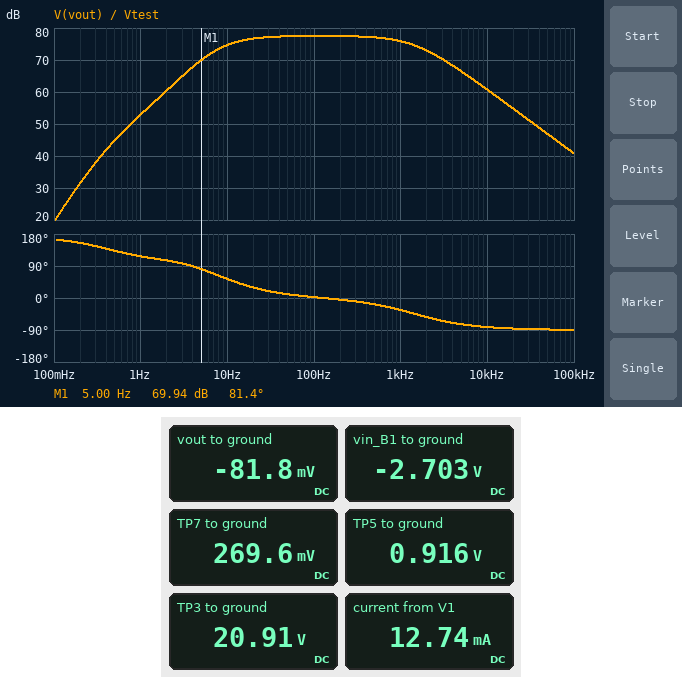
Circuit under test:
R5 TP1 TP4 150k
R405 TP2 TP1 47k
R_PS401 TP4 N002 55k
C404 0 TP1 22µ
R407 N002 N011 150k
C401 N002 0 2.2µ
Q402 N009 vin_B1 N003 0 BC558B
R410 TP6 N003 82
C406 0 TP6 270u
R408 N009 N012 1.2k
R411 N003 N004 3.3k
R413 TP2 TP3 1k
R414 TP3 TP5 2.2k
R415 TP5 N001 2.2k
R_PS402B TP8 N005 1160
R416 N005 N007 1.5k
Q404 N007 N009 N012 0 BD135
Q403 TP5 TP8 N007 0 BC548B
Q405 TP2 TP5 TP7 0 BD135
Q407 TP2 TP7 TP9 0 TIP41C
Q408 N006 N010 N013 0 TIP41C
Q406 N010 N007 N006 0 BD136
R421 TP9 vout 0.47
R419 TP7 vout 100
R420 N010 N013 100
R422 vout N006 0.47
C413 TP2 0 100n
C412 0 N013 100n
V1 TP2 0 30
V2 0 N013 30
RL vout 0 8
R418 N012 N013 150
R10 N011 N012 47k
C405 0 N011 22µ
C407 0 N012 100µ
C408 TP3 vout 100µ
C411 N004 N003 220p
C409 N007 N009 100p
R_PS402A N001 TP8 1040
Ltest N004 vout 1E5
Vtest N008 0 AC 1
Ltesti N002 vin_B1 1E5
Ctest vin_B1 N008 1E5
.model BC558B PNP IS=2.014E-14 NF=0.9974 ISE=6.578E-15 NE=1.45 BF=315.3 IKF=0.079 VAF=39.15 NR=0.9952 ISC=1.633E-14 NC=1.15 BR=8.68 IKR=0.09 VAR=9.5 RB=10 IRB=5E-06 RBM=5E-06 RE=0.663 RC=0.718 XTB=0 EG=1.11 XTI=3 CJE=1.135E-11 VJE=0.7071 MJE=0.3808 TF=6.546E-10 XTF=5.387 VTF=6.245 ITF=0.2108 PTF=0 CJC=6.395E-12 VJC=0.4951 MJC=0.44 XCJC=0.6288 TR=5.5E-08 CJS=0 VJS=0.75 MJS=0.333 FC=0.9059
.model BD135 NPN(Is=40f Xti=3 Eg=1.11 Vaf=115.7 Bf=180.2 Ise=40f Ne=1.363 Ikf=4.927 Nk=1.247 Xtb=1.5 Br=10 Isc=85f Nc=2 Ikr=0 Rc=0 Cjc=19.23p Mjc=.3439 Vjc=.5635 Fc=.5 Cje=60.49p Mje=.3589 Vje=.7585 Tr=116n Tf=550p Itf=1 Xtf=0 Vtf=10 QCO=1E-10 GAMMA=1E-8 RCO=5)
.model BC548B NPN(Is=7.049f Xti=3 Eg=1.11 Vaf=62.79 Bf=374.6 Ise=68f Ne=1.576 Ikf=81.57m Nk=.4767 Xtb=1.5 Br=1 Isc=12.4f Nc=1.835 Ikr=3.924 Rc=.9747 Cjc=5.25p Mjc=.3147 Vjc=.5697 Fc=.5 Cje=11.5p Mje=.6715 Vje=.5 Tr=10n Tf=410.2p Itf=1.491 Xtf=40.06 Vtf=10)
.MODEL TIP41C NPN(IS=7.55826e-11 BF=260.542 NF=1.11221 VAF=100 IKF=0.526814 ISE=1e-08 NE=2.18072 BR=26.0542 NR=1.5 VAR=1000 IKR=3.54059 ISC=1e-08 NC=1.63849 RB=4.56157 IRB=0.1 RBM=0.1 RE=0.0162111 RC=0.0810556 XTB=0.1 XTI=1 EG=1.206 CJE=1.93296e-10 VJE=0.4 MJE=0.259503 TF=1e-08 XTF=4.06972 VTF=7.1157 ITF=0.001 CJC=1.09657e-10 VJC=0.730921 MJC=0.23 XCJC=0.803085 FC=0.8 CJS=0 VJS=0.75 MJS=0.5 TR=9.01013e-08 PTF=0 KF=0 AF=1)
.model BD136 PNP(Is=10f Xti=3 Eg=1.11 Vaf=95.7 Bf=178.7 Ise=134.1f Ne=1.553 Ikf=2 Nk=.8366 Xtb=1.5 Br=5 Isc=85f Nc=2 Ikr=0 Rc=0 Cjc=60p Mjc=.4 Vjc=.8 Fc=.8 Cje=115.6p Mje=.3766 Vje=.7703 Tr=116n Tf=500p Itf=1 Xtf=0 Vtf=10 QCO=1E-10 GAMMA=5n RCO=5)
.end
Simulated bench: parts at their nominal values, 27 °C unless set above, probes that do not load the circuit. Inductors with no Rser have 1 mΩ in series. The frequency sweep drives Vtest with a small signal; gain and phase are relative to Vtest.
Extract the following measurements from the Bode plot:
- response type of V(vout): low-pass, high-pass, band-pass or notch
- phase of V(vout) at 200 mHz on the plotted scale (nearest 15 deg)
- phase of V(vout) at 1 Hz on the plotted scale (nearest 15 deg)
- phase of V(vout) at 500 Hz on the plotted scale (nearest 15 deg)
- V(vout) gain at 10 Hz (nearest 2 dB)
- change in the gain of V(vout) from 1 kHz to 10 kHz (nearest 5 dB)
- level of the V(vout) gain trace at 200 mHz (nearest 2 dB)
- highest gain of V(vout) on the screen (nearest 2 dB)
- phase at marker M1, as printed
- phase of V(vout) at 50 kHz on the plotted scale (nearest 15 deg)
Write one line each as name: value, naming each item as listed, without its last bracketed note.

response type of V(vout): low-pass, high-pass, band-pass or notch: band-pass
phase of V(vout) at 200 mHz on the plotted scale: 150 deg
phase of V(vout) at 1 Hz on the plotted scale: 120 deg
phase of V(vout) at 500 Hz on the plotted scale: -15 deg
V(vout) gain at 10 Hz: 74 dB
change in the gain of V(vout) from 1 kHz to 10 kHz: -15 dB
level of the V(vout) gain trace at 200 mHz: 32 dB
highest gain of V(vout) on the screen: 78 dB
phase at marker M1, as printed: 81.4 deg
phase of V(vout) at 50 kHz on the plotted scale: -90 deg
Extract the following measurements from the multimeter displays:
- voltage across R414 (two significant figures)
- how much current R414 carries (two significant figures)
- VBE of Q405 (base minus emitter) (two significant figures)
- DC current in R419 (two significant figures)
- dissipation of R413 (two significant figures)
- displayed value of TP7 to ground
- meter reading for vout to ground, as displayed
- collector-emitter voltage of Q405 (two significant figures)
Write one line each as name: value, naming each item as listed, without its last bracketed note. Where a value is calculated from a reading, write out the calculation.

voltage across R414: 20.91 V - 916 mV = 20 V
how much current R414 carries: (20.91 V - 916 mV) / 2.2 kΩ = 9.1 mA
VBE of Q405 (base minus emitter): 916 mV - 269.6 mV = 650 mV
DC current in R419: (269.6 mV - (-81.8 mV)) / 100 Ω = 3.5 mA
dissipation of R413: (30 V - 20.91 V)^2 / 1 kΩ = 83 mW
displayed value of TP7 to ground: 269.6 mV
meter reading for vout to ground, as displayed: -81.8 mV
collector-emitter voltage of Q405: 30 V - 269.6 mV = 30 V
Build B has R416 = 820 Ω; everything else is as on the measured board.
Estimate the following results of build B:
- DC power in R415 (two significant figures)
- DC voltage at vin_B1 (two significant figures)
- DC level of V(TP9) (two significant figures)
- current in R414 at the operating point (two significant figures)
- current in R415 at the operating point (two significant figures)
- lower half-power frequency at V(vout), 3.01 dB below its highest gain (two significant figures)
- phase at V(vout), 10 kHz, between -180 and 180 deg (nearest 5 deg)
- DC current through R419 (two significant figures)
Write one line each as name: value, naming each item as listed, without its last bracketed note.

DC power in R415: 340 µW
DC voltage at vin_B1: -2.7 V
DC level of V(TP9): -69 mV
current in R414 at the operating point: 9.0 mA
current in R415 at the operating point: 390 µA
lower half-power frequency at V(vout), 3.01 dB below its highest gain: 12 Hz
phase at V(vout), 10 kHz, between -180 and 180 deg: -85 deg
DC current through R419: 6.0 mA
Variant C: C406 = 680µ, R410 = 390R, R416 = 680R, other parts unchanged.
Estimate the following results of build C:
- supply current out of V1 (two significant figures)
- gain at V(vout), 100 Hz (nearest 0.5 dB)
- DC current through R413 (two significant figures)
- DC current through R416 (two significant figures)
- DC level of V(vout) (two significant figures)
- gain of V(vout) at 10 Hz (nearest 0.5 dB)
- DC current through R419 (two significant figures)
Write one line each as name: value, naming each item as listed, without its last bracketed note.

supply current out of V1: 120 mA
gain at V(vout), 100 Hz: 70.5 dB
DC current through R413: 9.0 mA
DC current through R416: 390 µA
DC level of V(vout): -94 mV
gain of V(vout) at 10 Hz: 67.0 dB
DC current through R419: 6.6 mA
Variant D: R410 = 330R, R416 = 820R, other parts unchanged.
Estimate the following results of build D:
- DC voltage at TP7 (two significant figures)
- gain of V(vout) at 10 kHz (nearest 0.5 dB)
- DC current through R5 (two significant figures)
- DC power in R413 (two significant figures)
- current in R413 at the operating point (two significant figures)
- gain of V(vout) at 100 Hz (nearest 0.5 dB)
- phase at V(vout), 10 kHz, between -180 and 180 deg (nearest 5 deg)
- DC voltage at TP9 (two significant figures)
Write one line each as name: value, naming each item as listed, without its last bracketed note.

DC voltage at TP7: 510 mV
gain of V(vout) at 10 kHz: 51.5 dB
DC current through R5: 130 µA
DC power in R413: 81 mW
current in R413 at the operating point: 9.0 mA
gain of V(vout) at 100 Hz: 71.5 dB
phase at V(vout), 10 kHz, between -180 and 180 deg: -85 deg
DC voltage at TP9: -69 mV
